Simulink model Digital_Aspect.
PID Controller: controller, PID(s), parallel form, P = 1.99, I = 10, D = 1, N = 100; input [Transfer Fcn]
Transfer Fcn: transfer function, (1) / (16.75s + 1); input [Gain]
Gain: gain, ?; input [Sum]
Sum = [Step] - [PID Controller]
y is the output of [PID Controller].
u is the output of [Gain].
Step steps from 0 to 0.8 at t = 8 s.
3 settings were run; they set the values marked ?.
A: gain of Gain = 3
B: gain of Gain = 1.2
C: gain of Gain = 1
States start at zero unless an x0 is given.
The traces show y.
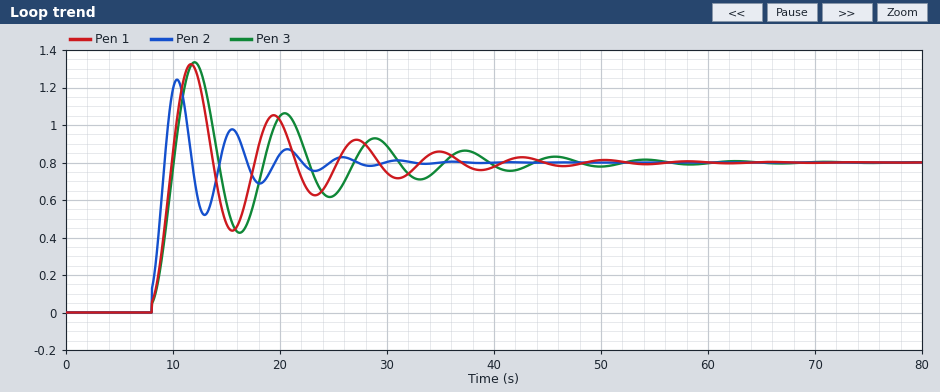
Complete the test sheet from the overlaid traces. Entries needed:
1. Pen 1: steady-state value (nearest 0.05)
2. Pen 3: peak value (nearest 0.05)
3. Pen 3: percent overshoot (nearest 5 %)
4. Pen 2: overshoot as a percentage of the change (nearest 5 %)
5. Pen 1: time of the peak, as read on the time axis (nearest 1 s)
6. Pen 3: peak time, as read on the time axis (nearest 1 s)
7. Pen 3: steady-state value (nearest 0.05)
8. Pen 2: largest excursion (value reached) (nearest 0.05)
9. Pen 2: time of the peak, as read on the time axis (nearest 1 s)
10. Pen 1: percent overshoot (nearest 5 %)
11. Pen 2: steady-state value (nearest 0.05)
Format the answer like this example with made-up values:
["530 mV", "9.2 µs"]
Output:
["0.80", "1.35", "65 %", "55 %", "12 s", "12 s", "0.80", "1.25", "10 s", "65 %", "0.80"]
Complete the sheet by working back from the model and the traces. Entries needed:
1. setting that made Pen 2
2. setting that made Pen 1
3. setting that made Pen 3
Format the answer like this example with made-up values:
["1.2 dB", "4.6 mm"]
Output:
["A", "B", "C"]
